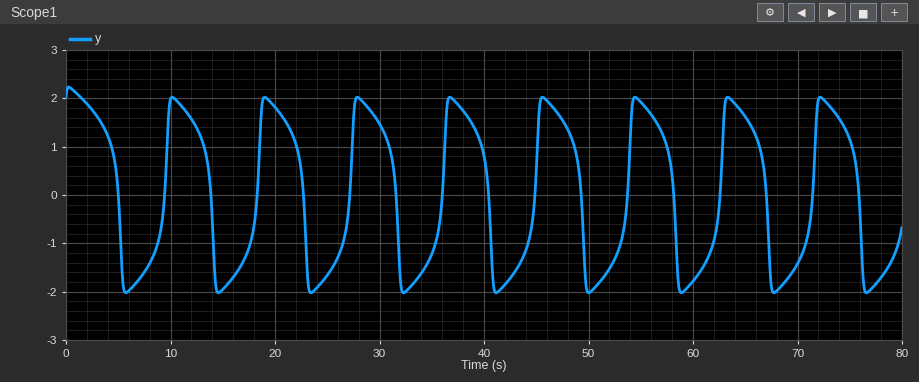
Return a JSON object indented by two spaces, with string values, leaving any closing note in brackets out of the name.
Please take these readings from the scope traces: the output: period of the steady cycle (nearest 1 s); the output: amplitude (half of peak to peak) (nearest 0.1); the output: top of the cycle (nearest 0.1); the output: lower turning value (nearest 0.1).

{
  "the output: period of the steady cycle": "9 s",
  "the output: amplitude (half of peak to peak)": "2.0",
  "the output: top of the cycle": "2.0",
  "the output: lower turning value": "-2.0"
}
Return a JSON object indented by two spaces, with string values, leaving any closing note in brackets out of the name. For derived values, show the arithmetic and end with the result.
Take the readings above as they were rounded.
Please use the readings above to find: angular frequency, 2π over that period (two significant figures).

{
  "angular frequency, 2π over that period": "2π / 9 = 0.70 rad/s"
}
